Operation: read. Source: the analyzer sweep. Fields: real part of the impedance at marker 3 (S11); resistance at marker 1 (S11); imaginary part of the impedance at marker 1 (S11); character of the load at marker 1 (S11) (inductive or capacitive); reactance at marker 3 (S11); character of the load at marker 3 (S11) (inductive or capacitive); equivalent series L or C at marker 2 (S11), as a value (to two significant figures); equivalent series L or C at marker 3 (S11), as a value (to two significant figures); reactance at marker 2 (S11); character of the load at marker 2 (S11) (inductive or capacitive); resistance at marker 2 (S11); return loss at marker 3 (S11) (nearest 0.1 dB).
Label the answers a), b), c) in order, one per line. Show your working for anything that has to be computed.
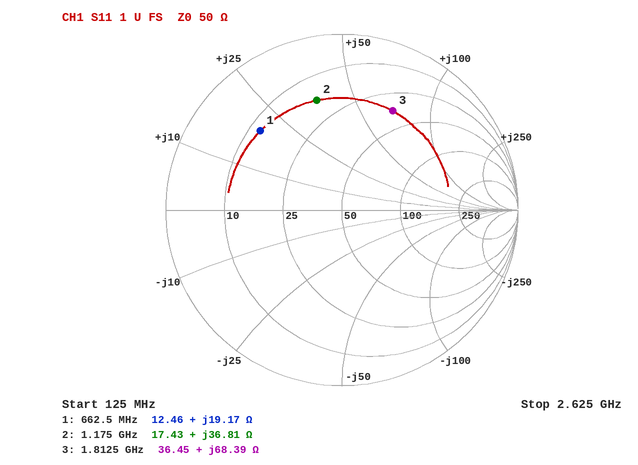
a) 36.45 Ω
b) 12.46 Ω
c) +19.17 Ω
d) inductive
e) +68.39 Ω
f) inductive
g) L = 36.81 Ω/(2π × 1.175 GHz) ≈ 5.0 nH
h) L = 68.39 Ω/(2π × 1.8125 GHz) ≈ 6.0 nH
i) +36.81 Ω
j) inductive
k) 17.43 Ω
l) 4.0 dB
